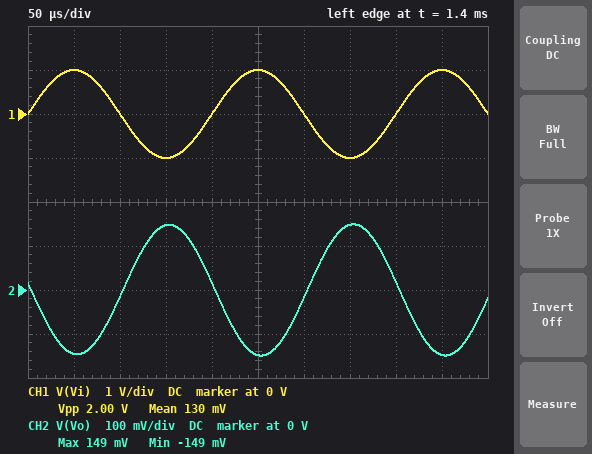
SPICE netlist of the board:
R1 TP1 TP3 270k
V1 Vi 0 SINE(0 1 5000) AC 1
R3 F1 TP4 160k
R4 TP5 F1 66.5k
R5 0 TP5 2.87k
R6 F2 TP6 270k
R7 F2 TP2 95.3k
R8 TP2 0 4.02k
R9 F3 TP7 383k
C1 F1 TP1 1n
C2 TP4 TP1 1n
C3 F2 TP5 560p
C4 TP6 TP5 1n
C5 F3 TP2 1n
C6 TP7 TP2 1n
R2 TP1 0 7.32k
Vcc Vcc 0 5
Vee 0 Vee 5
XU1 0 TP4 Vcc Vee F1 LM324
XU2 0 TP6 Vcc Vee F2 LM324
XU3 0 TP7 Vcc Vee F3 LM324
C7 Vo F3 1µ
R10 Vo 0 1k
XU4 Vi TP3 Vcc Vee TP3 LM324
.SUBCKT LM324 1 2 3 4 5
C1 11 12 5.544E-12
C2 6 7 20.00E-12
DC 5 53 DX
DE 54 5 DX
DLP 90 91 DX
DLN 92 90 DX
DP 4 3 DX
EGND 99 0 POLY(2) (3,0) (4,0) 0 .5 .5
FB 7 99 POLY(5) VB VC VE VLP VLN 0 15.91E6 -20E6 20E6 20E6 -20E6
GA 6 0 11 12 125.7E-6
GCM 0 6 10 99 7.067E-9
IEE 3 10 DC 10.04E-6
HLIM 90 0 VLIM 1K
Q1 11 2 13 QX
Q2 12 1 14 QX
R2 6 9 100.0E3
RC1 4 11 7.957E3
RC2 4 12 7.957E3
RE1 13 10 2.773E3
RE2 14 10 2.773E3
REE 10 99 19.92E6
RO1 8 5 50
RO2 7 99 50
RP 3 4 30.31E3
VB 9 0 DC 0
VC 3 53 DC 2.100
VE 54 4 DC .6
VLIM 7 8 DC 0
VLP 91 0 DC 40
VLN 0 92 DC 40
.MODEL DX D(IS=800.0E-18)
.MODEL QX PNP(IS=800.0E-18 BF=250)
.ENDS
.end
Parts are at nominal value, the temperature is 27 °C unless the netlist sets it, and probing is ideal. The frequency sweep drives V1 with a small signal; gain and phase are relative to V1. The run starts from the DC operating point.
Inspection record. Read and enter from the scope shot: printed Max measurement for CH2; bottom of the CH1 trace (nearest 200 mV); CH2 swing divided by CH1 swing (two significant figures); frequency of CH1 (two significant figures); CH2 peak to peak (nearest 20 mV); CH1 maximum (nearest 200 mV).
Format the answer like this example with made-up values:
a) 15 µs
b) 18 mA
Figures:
a) 149 mV
b) -1.0 V
c) 0.15
d) 5.0 kHz
e) 300 mV
f) 1.0 V
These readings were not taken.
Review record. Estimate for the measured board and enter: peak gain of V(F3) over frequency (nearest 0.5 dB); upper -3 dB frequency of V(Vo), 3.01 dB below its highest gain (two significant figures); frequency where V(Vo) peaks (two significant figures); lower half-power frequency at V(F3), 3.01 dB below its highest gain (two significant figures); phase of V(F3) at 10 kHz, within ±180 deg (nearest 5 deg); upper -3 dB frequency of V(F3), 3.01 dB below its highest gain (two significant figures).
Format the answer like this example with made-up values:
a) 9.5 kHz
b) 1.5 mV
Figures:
a) -13.5 dB
b) 5.0 kHz
c) 4.2 kHz
d) 3.9 kHz
e) -55 deg
f) 5.0 kHz
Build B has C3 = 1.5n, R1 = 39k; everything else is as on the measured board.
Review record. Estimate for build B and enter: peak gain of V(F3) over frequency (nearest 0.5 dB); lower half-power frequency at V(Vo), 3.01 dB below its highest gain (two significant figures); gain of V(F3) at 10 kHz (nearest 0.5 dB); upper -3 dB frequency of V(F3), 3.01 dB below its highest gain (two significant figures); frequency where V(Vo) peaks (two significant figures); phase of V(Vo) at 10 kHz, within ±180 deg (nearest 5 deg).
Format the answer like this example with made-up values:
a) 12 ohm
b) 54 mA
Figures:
a) 11.5 dB
b) 4.1 kHz
c) -34.5 dB
d) 4.9 kHz
e) 4.5 kHz
f) -65 deg
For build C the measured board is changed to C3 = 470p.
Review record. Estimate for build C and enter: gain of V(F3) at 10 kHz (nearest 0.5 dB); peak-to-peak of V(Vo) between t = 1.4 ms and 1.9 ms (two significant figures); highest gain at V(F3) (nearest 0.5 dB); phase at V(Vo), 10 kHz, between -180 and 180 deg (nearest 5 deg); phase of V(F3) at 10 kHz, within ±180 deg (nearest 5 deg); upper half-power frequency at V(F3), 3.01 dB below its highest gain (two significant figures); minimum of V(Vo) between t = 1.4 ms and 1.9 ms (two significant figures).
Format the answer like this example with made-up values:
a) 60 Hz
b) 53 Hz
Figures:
a) -36.0 dB
b) 270 mV
c) -14.0 dB
d) -45 deg
e) -50 deg
f) 4.9 kHz
g) -130 mV
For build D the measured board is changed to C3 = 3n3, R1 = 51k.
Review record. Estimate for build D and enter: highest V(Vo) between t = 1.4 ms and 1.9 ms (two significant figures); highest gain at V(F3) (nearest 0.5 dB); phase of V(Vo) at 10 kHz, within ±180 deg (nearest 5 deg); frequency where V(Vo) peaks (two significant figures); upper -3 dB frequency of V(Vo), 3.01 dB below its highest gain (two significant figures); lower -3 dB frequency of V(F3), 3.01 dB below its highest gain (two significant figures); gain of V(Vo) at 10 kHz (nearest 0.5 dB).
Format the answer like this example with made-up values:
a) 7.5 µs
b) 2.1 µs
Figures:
a) 320 mV
b) -0.5 dB
c) -65 deg
d) 4.0 kHz
e) 4.4 kHz
f) 3.5 kHz
g) -44.5 dB
